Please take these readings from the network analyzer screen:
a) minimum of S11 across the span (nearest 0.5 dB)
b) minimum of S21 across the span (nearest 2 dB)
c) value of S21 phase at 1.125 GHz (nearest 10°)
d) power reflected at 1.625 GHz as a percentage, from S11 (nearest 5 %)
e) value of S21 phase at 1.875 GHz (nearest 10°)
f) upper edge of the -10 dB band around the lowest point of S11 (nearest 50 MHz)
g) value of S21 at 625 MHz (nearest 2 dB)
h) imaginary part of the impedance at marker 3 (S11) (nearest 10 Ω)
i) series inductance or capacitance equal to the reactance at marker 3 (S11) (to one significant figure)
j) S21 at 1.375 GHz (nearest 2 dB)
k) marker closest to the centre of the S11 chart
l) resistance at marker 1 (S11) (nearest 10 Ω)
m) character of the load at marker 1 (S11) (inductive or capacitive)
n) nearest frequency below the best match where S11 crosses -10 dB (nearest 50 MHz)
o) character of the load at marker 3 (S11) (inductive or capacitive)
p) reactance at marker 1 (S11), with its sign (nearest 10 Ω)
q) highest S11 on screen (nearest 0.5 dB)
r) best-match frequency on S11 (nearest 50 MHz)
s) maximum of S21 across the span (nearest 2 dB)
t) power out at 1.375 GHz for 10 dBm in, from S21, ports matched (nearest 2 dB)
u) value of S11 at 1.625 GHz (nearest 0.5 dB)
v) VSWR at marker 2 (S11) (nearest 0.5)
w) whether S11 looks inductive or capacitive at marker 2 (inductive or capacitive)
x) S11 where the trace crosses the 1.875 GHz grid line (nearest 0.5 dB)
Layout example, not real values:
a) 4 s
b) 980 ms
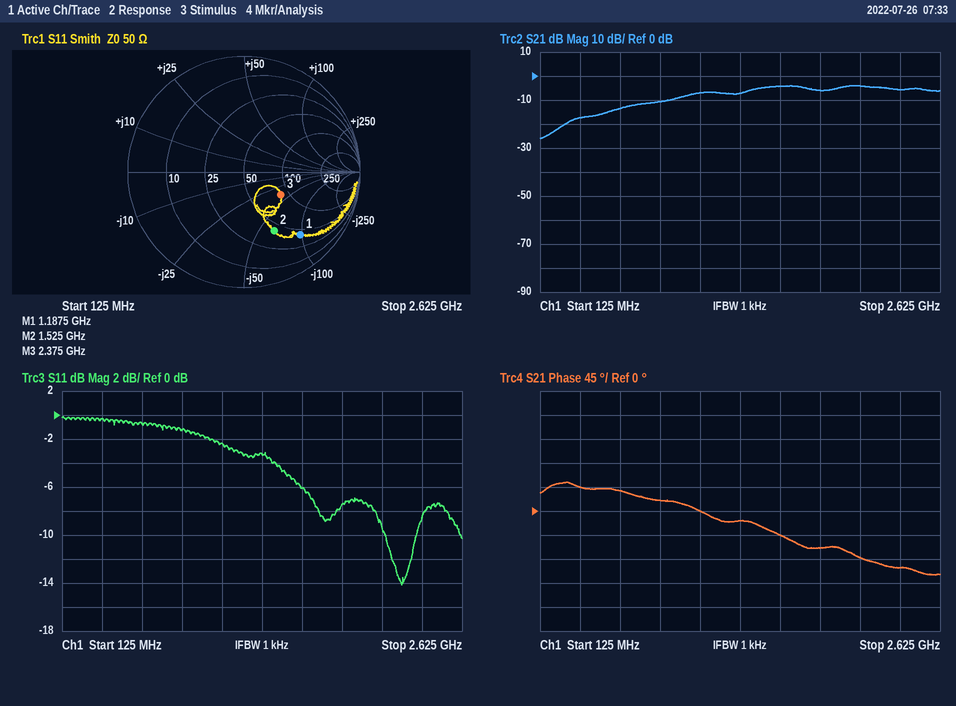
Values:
a) -14.0 dB
b) -26 dB
c) 0°
d) 25 %
e) -70°
f) 2.35 GHz
g) -14 dB
h) -40 Ω
i) 2 pF
j) -8 dB
k) marker 3
l) 40 Ω
m) capacitive
n) 2.15 GHz
o) capacitive
p) -100 Ω
q) 0.0 dB
r) 2.25 GHz
s) -4 dB
t) 2 dBm
u) -6.0 dB
v) 3.5
w) capacitive
x) -7.5 dB
